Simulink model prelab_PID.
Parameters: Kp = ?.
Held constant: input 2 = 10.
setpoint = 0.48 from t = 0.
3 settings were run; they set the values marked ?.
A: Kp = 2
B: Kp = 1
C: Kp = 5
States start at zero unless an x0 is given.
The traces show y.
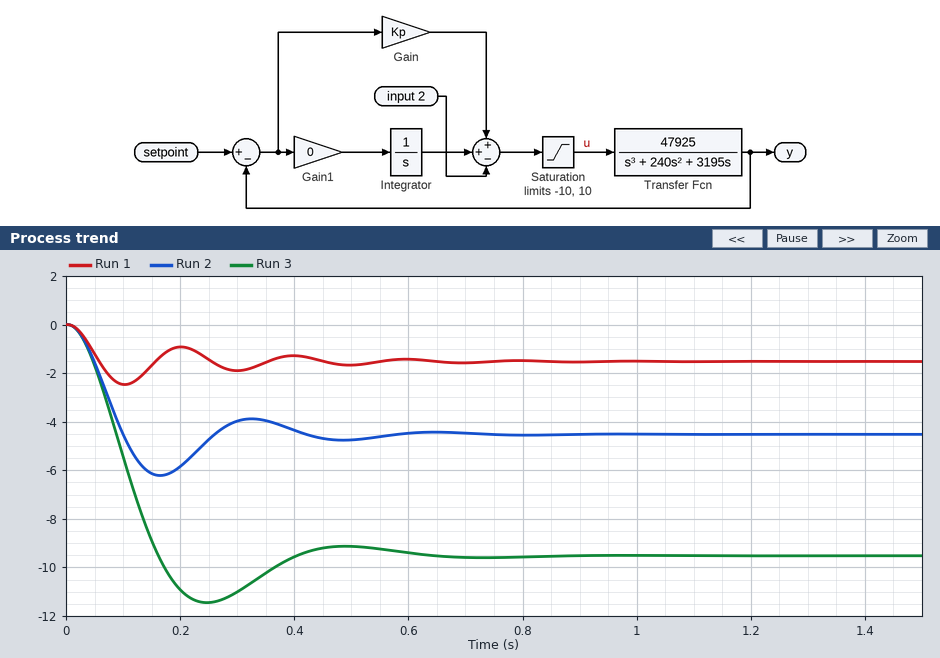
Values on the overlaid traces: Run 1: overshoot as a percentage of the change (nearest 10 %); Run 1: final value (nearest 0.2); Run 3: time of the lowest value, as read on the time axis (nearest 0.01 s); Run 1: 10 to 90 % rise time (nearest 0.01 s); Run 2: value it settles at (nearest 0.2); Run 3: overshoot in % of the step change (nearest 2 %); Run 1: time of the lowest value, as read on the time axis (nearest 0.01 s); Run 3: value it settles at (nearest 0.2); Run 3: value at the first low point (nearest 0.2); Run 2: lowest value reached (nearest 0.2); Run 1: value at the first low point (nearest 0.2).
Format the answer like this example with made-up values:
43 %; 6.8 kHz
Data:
60 %; -1.6; 0.25 s; 0.04 s; -4.6; 20 %; 0.10 s; -9.6; -11.4; -6.2; -2.4
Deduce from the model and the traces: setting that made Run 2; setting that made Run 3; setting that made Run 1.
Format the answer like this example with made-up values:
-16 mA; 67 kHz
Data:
A; B; C
